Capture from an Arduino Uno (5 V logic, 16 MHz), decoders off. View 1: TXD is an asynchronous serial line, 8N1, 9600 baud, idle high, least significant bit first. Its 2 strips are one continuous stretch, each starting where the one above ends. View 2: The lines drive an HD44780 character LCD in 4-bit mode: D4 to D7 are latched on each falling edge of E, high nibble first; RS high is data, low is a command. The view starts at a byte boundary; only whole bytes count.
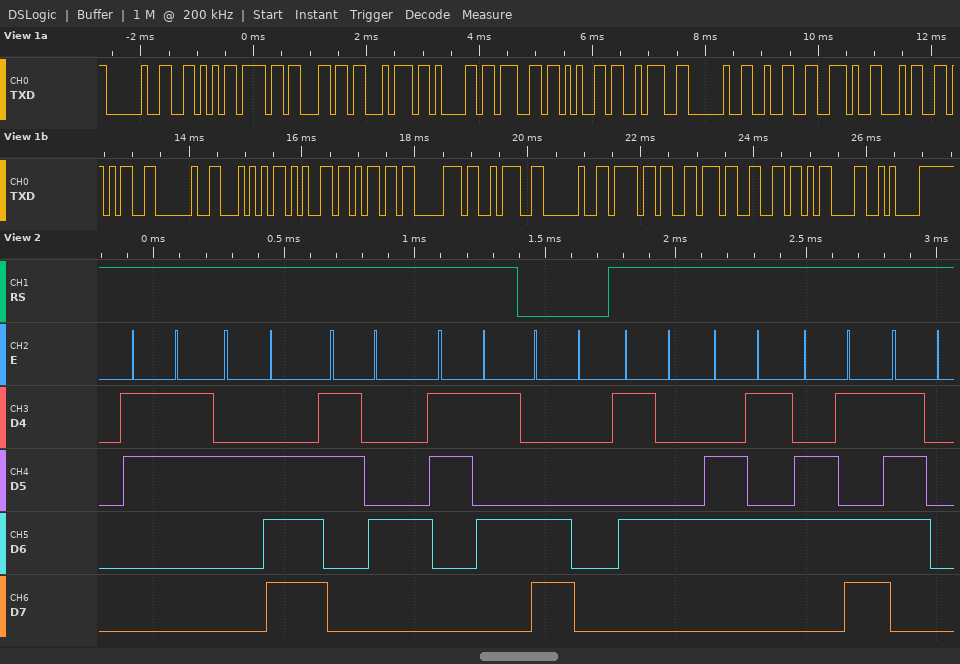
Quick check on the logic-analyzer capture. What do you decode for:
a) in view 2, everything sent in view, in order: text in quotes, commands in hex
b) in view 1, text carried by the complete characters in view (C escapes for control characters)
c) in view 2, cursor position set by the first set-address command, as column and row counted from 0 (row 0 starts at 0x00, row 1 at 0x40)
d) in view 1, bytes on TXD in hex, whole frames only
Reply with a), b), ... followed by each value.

a) "3.45" 0xC0 "Temp"
b) " Voltage: 2.45 Temp: ovf\r\n"
c) column 0, row 1
d) 20 56 6F 6C 74 61 67 65 3A 20 32 2E 34 35 20 54 65 6D 70 3A 20 6F 76 66 0D 0A
